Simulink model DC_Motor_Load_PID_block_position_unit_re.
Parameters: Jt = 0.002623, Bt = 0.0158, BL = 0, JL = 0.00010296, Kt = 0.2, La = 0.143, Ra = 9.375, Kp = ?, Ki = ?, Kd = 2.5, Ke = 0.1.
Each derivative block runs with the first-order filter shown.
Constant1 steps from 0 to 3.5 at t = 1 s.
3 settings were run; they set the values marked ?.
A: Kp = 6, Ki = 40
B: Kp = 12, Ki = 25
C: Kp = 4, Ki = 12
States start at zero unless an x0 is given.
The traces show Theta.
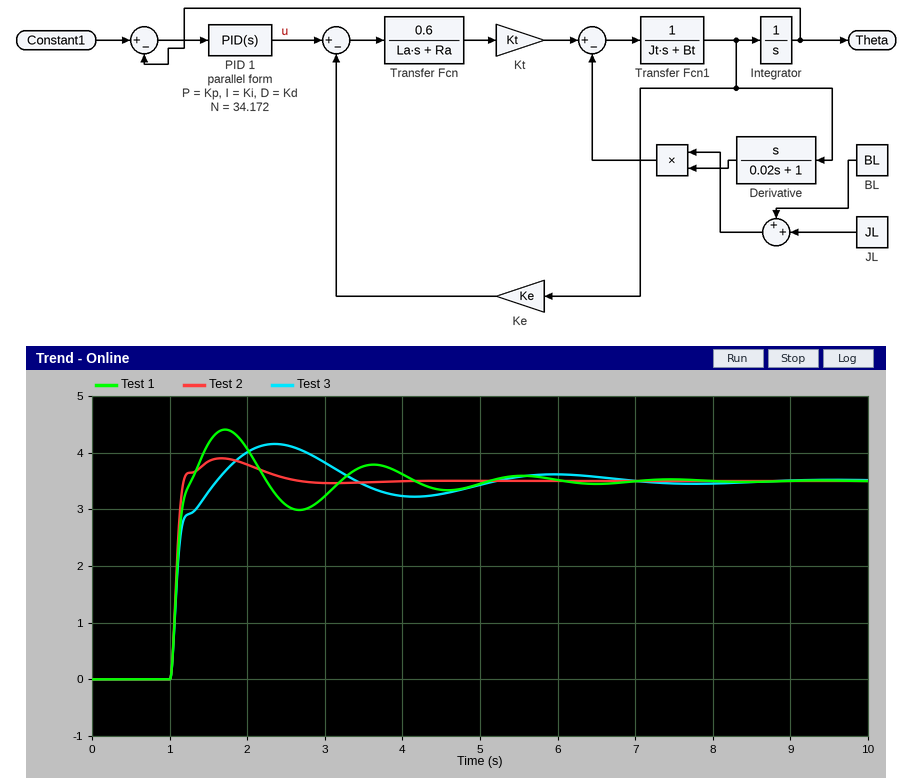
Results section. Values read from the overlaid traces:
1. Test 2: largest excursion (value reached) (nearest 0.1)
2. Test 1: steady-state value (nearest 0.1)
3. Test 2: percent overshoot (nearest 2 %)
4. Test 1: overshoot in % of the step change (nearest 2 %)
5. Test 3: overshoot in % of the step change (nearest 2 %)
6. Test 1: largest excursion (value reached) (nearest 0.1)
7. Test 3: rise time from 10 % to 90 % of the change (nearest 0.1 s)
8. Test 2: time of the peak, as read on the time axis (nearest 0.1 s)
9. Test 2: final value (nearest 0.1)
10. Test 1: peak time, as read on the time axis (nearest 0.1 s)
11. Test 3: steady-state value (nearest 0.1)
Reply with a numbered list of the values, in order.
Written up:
1. 3.9
2. 3.5
3. 12 %
4. 26 %
5. 18 %
6. 4.4
7. 0.4 s
8. 1.7 s
9. 3.5
10. 1.7 s
11. 3.5
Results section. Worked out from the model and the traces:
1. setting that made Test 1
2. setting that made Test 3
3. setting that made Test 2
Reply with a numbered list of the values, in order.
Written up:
1. A
2. C
3. B
